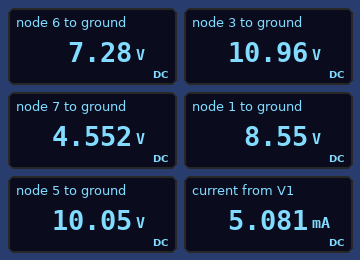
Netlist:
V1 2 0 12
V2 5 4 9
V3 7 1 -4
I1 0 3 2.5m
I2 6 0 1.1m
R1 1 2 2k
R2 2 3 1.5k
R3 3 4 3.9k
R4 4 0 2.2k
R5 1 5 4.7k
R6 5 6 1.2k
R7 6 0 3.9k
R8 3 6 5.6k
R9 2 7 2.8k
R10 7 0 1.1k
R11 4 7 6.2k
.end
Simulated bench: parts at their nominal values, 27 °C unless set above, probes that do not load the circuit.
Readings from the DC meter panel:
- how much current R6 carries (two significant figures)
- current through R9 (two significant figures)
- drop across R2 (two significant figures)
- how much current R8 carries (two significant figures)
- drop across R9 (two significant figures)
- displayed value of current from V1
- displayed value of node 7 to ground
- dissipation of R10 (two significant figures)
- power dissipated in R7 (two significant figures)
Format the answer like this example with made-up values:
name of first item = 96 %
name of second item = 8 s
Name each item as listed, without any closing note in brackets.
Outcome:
how much current R6 carries = 2.3 mA
current through R9 = 2.7 mA
drop across R2 = 1.0 V
how much current R8 carries = 660 µA
drop across R9 = 7.4 V
displayed value of current from V1 = 5.081 mA
displayed value of node 7 to ground = 4.552 V
dissipation of R10 = 19 mW
power dissipated in R7 = 14 mW
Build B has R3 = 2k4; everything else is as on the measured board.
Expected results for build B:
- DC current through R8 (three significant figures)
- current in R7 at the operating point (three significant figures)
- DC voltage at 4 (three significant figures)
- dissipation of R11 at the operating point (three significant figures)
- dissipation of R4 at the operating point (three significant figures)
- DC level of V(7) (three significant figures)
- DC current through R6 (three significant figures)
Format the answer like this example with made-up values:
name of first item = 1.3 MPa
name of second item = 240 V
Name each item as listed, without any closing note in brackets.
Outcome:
DC current through R8 = 422 µA
current in R7 at the operating point = 1.95 mA
DC voltage at 4 = 1.78 V
dissipation of R11 at the operating point = 1.36 mW
dissipation of R4 at the operating point = 1.44 mW
DC level of V(7) = 4.68 V
DC current through R6 = 2.63 mA
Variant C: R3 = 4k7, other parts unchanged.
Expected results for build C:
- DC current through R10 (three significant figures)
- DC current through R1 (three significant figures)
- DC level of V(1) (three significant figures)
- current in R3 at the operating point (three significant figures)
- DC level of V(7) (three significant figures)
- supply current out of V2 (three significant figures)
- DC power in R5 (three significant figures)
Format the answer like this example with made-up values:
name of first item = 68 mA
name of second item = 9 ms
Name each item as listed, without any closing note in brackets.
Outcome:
DC current through R10 = 4.10 mA
DC current through R1 = 1.75 mA
DC level of V(1) = 8.51 V
current in R3 at the operating point = 2.23 mA
DC level of V(7) = 4.51 V
supply current out of V2 = 2.47 mA
DC power in R5 = 353 µW
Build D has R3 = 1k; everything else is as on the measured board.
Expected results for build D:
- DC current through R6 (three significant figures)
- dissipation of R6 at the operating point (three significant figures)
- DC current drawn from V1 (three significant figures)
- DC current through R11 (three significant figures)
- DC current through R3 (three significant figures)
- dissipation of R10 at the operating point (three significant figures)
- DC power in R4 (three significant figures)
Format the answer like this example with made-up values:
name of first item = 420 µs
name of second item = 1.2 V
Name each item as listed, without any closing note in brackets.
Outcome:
DC current through R6 = 3.23 mA
dissipation of R6 at the operating point = 12.5 mW
DC current drawn from V1 = 6.61 mA
DC current through R11 = 287 µA
DC current through R3 = 5.05 mA
dissipation of R10 at the operating point = 22.0 mW
DC power in R4 = 4.47 mW
